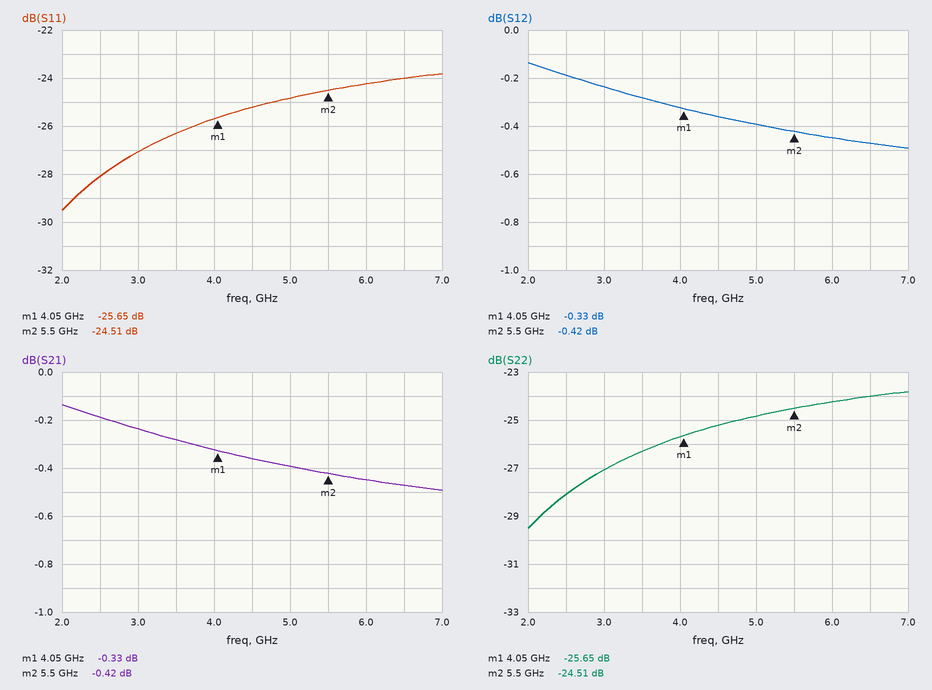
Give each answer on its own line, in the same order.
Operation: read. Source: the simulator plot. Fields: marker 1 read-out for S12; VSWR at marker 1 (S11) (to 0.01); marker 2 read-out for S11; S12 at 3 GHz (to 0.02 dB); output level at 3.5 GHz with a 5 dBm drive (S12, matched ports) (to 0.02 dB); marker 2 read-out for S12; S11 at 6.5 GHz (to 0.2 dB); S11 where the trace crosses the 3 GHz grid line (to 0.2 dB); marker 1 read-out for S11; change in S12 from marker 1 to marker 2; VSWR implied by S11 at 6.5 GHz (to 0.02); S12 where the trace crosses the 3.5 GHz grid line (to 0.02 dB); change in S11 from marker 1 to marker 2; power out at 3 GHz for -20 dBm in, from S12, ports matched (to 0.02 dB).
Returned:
-0.33 dB
1.11
-24.51 dB
-0.24 dB
4.72 dBm
-0.42 dB
-24.0 dB
-27.0 dB
-25.65 dB
-0.09 dB
1.14
-0.28 dB
1.14 dB
-20.24 dBm
